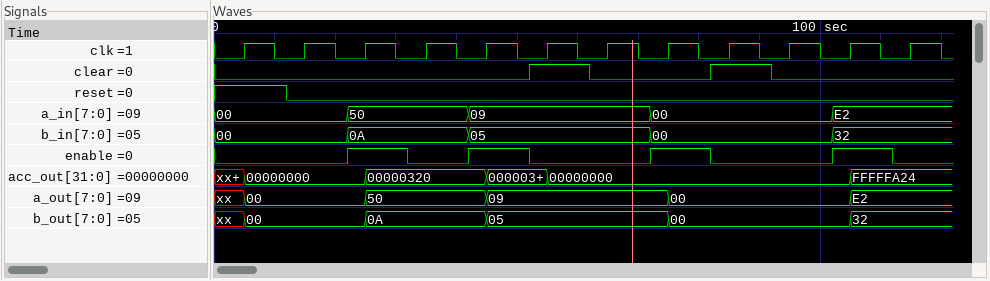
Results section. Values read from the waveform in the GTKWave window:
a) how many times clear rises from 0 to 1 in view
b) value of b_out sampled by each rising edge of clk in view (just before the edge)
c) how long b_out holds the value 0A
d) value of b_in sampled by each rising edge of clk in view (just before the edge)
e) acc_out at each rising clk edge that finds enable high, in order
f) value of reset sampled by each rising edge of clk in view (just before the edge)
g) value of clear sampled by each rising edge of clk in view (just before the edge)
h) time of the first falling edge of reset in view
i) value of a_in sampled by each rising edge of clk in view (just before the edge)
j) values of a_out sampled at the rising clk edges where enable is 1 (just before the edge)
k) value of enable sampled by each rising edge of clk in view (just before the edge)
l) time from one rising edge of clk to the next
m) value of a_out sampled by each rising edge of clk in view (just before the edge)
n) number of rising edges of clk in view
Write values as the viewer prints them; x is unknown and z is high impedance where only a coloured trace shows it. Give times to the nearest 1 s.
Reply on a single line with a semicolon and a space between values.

2; xx, 00, 00, 0A, 0A, 05, 05, 05, 00, 00, 00, 32; 20 s; 00, 00, 0A, 0A, 05, 05, 05, 00, 00, 00, 32, 32; 00000000, 00000320, 00000000, 00000000; 1 0 0 0 0 0 0 0 0 0 0 0; 0 0 0 0 0 1 0 0 1 0 0 0; 12 s; 00, 00, 50, 50, 09, 09, 09, 00, 00, 00, E2, E2; 00, 50, 09, 00; 0 0 1 0 1 0 0 1 0 0 1 0; 10 s; xx, 00, 00, 50, 50, 09, 09, 09, 00, 00, 00, E2; 12
